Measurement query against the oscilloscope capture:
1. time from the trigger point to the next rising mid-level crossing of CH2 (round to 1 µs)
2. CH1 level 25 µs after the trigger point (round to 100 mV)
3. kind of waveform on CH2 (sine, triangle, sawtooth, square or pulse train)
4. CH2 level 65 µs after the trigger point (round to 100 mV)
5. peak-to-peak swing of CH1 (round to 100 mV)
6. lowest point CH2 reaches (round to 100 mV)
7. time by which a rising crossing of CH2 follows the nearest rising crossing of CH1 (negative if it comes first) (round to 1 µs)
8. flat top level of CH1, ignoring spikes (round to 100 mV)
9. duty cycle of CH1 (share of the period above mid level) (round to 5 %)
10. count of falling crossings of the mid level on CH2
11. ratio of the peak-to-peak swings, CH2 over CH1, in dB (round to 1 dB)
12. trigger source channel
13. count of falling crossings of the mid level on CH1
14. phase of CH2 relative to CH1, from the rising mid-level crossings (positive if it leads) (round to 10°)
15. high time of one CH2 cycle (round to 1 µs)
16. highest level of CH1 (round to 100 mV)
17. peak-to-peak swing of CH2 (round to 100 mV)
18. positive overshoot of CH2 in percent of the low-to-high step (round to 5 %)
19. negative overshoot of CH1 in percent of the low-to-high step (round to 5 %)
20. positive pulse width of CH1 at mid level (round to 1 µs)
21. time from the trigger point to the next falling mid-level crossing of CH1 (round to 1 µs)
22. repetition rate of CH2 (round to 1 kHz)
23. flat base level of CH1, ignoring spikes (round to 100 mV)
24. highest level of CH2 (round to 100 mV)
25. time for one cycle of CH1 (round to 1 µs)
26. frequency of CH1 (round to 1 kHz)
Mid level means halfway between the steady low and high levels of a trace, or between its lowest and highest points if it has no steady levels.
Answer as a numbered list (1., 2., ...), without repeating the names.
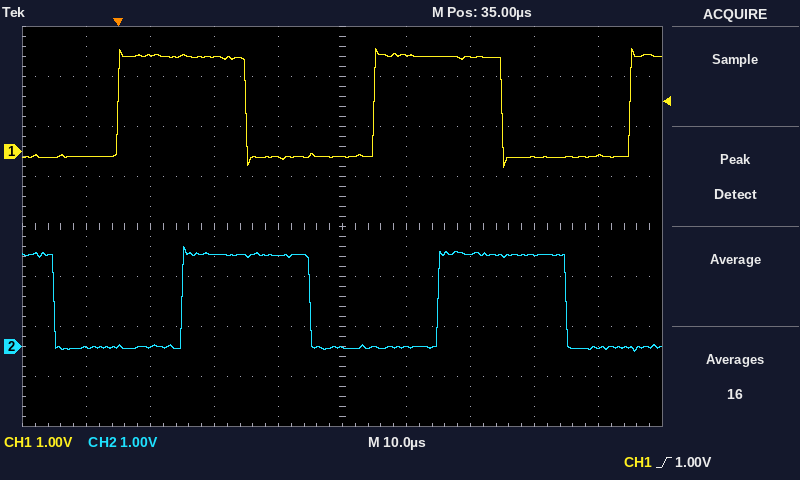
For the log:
1. 10 µs
2. -100 mV
3. square
4. 1.8 V
5. 2.4 V
6. -100 mV
7. +10 µs
8. 1.9 V
9. 50 %
10. 3
11. -1 dB
12. CH1
13. 2
14. -90°
15. 20 µs
16. 2.1 V
17. 2.1 V
18. 10 %
19. 10 %
20. 20 µs
21. 20 µs
22. 25 kHz
23. -100 mV
24. 2.0 V
25. 40 µs
26. 25 kHz
